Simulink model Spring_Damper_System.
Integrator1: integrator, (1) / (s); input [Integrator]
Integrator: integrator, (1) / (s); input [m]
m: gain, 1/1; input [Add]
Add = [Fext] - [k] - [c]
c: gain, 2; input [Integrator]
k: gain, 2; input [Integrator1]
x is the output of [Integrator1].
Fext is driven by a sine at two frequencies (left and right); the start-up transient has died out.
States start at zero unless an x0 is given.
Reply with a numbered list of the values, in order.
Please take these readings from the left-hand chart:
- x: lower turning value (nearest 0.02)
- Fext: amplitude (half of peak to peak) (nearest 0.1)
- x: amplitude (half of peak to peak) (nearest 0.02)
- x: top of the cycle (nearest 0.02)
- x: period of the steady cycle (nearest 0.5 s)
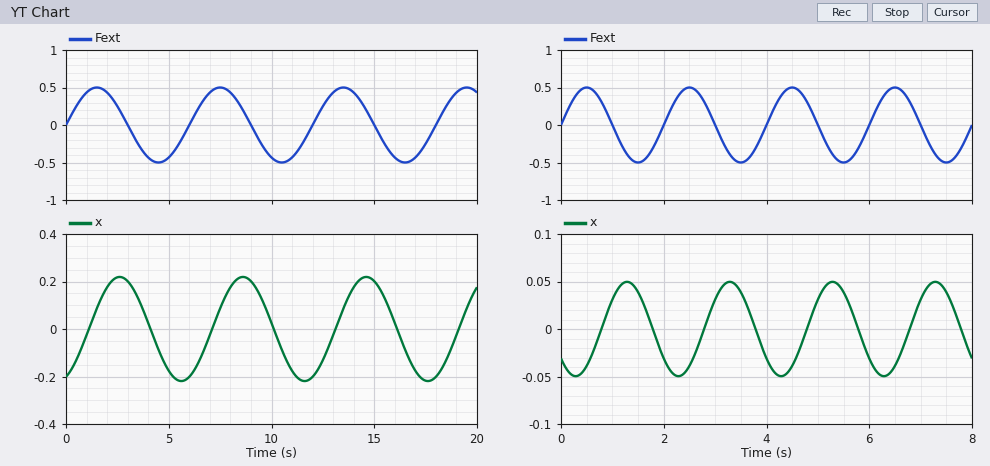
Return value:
1. -0.22
2. 0.5
3. 0.22
4. 0.22
5. 6.0 s
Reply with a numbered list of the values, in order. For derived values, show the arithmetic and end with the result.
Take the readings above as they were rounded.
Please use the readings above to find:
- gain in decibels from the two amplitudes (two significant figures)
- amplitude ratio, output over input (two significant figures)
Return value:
1. 20 log10(0.22 / 0.5) = -7.1 dB
2. 0.22 / 0.5 = 0.44
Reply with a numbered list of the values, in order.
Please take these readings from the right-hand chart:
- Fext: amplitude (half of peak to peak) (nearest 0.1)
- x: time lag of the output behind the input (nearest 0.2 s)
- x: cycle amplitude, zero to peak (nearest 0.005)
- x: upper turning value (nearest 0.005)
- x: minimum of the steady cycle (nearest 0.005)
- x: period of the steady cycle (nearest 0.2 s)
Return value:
1. 0.5
2. 0.8 s
3. 0.050
4. 0.050
5. -0.050
6. 2.0 s
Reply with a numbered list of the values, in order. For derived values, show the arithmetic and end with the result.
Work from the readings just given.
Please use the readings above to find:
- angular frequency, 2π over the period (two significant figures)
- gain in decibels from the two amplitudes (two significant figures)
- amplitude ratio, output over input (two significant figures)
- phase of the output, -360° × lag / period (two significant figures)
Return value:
1. 2π / 2 = 3.1 rad/s
2. 20 log10(0.05 / 0.5) = -20 dB
3. 0.05 / 0.5 = 0.10
4. -360 × 0.8 / 2 = -140°
